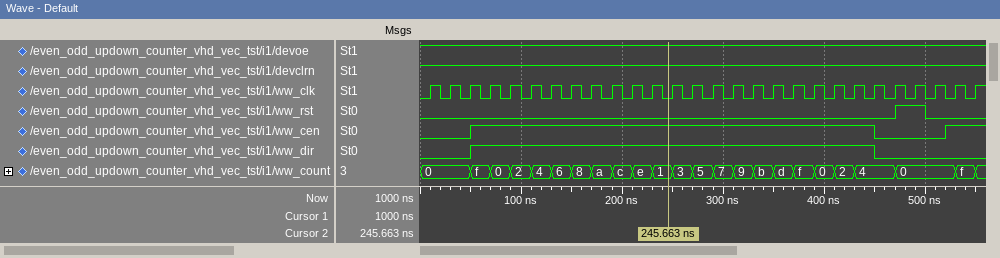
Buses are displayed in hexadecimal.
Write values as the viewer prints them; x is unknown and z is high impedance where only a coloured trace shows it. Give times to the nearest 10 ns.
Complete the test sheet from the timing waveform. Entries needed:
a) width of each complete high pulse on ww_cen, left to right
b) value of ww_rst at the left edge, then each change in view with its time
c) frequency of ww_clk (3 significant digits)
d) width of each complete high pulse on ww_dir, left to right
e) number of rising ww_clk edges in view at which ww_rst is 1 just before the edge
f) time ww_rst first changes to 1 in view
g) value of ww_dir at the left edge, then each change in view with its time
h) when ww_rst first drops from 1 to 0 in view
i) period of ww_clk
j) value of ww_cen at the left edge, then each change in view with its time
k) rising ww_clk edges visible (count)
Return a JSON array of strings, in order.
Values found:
["400 ns", "0, 1 at 470 ns, 0 at 500 ns", "50.0 MHz", "400 ns", "1", "470 ns", "0, 1 at 50 ns, 0 at 450 ns", "500 ns", "20 ns", "0, 1 at 50 ns, 0 at 450 ns, 1 at 520 ns", "28"]
